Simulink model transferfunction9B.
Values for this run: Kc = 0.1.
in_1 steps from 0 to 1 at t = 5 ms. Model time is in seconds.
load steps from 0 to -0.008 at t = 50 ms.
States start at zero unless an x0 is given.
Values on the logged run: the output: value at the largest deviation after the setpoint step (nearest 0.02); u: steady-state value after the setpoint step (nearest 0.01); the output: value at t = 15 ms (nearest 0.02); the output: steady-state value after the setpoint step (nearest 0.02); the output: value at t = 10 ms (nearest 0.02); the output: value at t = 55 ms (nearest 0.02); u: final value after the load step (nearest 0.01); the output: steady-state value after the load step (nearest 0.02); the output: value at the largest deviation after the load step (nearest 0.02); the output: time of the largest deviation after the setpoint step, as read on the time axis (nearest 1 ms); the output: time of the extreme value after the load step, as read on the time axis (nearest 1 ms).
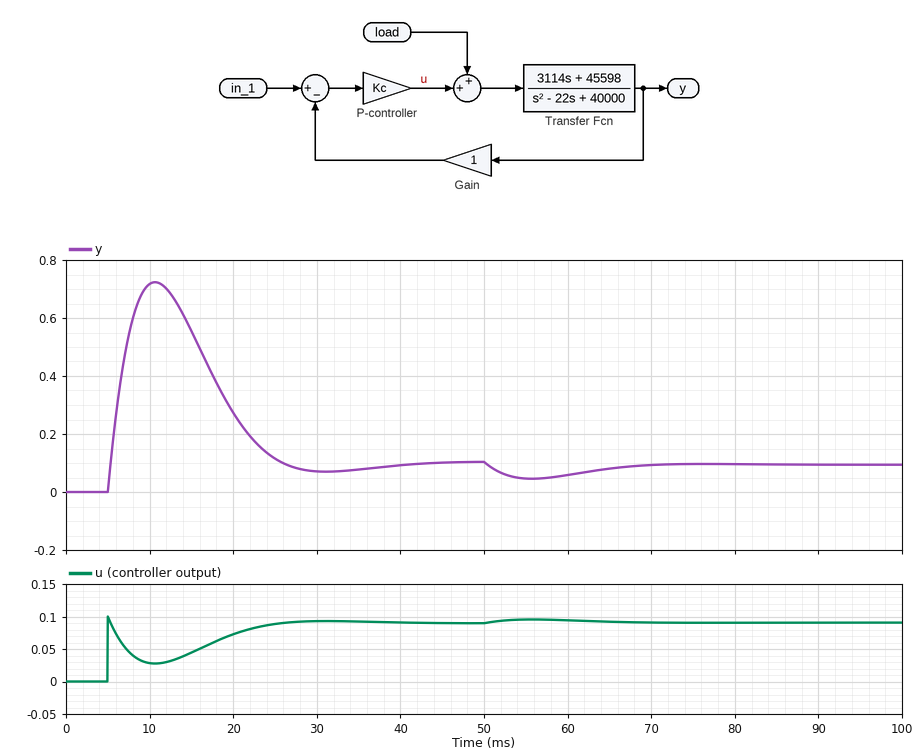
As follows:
0.72
0.09
0.56
0.10
0.72
0.04
0.09
0.10
0.04
11 ms
56 ms
